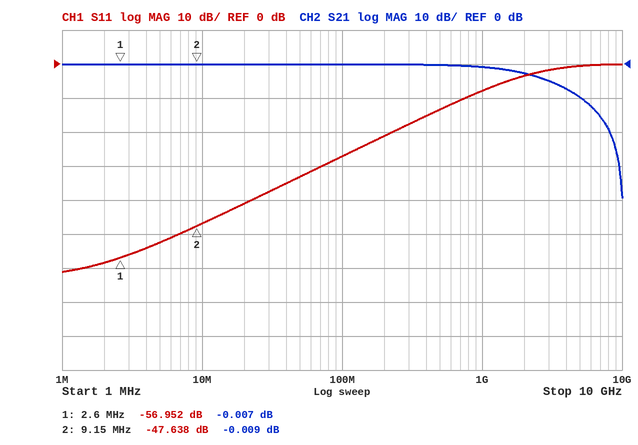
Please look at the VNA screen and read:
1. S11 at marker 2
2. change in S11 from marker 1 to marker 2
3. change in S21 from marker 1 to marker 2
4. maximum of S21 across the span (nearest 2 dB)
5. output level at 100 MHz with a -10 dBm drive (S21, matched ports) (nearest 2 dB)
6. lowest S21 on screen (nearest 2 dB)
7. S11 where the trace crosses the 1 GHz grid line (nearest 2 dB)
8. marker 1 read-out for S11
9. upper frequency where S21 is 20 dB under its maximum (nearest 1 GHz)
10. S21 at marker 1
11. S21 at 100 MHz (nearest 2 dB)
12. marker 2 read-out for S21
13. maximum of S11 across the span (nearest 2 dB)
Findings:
-47.638 dB
9.314 dB
-0.002 dB
0 dB
-10 dBm
-40 dB
-8 dB
-56.952 dB
8 GHz
-0.007 dB
0 dB
-0.009 dB
0 dB
